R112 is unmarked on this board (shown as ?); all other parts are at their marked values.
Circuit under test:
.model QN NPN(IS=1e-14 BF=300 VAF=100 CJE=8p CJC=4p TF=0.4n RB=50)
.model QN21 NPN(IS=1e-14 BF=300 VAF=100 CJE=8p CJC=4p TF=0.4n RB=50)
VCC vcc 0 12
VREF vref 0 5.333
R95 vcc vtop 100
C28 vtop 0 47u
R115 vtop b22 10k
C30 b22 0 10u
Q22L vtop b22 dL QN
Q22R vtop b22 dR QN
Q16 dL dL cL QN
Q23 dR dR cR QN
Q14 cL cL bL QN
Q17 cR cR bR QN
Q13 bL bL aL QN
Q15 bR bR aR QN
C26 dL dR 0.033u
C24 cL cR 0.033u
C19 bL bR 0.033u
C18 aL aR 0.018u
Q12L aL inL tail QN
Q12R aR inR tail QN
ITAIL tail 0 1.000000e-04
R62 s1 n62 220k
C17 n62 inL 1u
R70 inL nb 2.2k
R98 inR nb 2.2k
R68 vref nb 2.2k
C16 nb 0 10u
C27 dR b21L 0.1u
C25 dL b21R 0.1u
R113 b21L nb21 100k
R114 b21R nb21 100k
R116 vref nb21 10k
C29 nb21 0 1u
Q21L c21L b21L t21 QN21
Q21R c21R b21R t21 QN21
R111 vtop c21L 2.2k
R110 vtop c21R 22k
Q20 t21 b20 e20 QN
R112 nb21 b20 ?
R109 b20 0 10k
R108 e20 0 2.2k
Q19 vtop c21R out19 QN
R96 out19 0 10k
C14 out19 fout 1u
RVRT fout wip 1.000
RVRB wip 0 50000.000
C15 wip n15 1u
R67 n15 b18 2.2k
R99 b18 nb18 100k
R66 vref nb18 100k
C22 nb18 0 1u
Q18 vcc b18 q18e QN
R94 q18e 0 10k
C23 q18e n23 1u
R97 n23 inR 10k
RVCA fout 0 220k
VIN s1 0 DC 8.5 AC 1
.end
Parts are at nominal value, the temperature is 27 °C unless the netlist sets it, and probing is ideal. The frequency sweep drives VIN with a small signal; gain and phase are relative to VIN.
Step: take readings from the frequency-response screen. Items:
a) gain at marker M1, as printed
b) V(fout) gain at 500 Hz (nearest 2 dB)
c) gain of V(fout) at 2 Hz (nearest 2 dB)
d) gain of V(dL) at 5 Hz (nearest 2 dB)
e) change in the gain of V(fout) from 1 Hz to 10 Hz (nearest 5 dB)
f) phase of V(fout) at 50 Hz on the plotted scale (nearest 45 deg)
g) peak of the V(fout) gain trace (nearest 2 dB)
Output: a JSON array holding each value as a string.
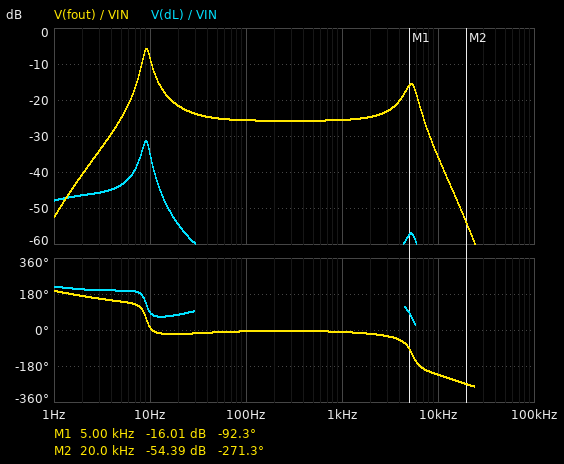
["-16.01 dB", "-26 dB", "-40 dB", "-44 dB", "45 dB", "0 deg", "-6 dB"]
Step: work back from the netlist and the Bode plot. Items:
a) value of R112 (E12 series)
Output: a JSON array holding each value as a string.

["22 kΩ"]
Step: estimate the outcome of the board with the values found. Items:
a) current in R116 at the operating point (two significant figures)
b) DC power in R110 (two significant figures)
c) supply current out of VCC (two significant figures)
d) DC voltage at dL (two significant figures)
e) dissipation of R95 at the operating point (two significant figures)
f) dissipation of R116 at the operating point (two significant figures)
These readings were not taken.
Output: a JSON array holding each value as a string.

["130 µA", "460 µW", "1.6 mA", "11 V", "140 µW", "160 µW"]
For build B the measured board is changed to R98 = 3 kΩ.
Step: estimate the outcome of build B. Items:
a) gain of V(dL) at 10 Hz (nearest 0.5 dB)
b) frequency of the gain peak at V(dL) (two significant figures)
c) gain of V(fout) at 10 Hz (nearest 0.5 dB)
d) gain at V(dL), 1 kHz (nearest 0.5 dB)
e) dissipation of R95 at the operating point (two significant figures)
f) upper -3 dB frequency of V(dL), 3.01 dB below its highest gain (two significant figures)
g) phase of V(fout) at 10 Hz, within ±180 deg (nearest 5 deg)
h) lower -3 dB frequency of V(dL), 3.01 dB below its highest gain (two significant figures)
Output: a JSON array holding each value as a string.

["-40.0 dB", "8.2 Hz", "-13.5 dB", "-69.0 dB", "140 µW", "8.5 Hz", "-20 deg", "7.8 Hz"]
